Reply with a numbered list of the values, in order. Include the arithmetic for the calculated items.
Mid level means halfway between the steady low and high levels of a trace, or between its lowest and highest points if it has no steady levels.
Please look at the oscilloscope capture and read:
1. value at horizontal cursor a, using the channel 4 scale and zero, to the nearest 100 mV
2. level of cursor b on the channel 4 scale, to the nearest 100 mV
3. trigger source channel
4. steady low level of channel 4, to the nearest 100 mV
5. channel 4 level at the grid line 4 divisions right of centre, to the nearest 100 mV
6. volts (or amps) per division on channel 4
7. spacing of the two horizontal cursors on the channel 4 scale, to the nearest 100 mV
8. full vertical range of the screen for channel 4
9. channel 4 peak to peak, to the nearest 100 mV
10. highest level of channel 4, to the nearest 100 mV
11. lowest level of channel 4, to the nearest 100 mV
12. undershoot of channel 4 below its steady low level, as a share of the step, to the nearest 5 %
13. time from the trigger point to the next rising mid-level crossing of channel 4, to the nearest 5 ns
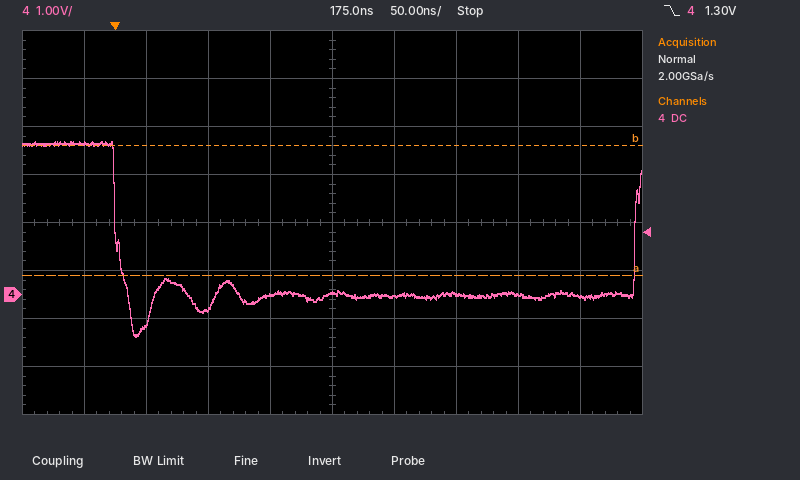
1. 400 mV
2. 3.1 V
3. channel 4
4. 0.0 V
5. 0.0 V
6. 1 V
7. 2.7 V
8. 8 V
9. 3.2 V − (-900 mV) = 4.1 V
10. 3.2 V
11. -900 mV
12. 25 %
13. 420 ns
